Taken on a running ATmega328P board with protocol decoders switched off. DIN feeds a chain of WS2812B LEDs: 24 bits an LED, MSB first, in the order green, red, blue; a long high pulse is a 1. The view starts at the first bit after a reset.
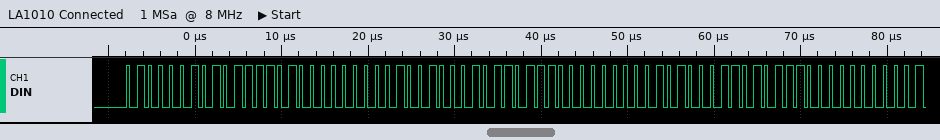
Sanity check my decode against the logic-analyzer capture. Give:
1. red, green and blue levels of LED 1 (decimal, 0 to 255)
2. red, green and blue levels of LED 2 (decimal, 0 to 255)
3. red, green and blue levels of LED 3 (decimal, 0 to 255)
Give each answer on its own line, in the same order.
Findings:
189, 66, 0
183, 72, 0
174, 81, 0
